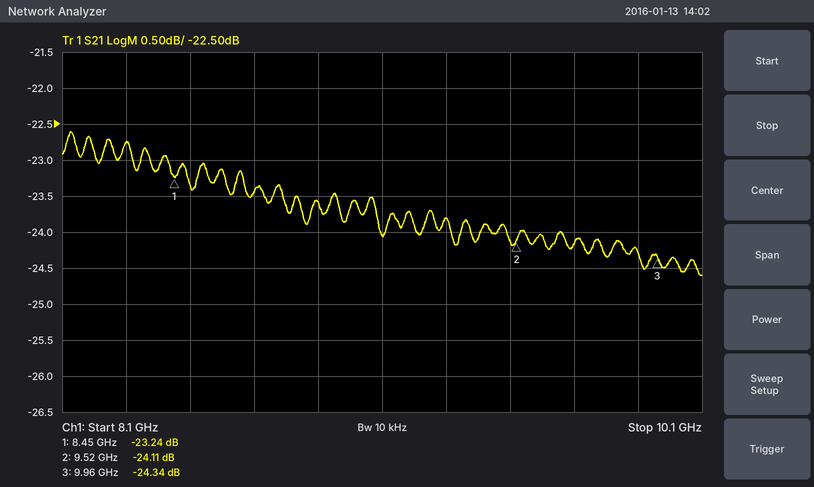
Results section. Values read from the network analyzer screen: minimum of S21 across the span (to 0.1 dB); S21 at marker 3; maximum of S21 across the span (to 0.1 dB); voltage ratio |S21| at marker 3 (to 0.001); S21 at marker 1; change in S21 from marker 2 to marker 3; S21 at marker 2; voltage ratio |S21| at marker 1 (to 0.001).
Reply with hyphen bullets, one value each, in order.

- -24.6 dB
- -24.34 dB
- -22.6 dB
- 0.061
- -23.24 dB
- -0.23 dB
- -24.11 dB
- 0.069
